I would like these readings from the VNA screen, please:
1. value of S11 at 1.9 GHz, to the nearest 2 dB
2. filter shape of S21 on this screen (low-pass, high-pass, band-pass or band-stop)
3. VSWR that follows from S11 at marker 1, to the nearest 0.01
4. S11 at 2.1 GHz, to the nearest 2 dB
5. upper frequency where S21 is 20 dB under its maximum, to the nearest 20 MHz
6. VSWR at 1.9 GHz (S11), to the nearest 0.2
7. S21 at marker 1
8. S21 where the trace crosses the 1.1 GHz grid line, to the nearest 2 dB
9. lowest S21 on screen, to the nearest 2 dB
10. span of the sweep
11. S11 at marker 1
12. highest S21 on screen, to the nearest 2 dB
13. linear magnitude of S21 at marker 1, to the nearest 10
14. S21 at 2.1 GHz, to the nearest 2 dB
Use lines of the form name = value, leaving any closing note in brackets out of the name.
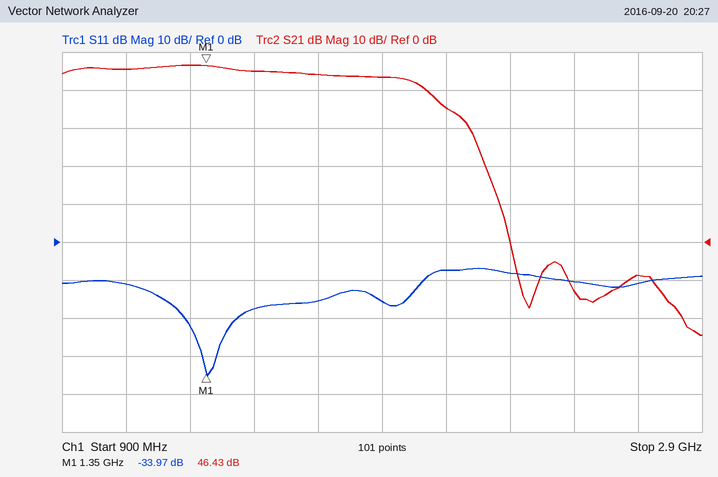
value of S11 at 1.9 GHz, to the nearest 2 dB = -16 dB
filter shape of S21 on this screen = low-pass
VSWR that follows from S11 at marker 1, to the nearest 0.01 = 1.04
S11 at 2.1 GHz, to the nearest 2 dB = -8 dB
upper frequency where S21 is 20 dB under its maximum, to the nearest 20 MHz = 2.20 GHz
VSWR at 1.9 GHz (S11), to the nearest 0.2 = 1.4
S21 at marker 1 = 46.43 dB
S21 where the trace crosses the 1.1 GHz grid line, to the nearest 2 dB = 46 dB
lowest S21 on screen, to the nearest 2 dB = -24 dB
span of the sweep = 2 GHz
S11 at marker 1 = -33.97 dB
highest S21 on screen, to the nearest 2 dB = 46 dB
linear magnitude of S21 at marker 1, to the nearest 10 = 210
S21 at 2.1 GHz, to the nearest 2 dB = 36 dB
